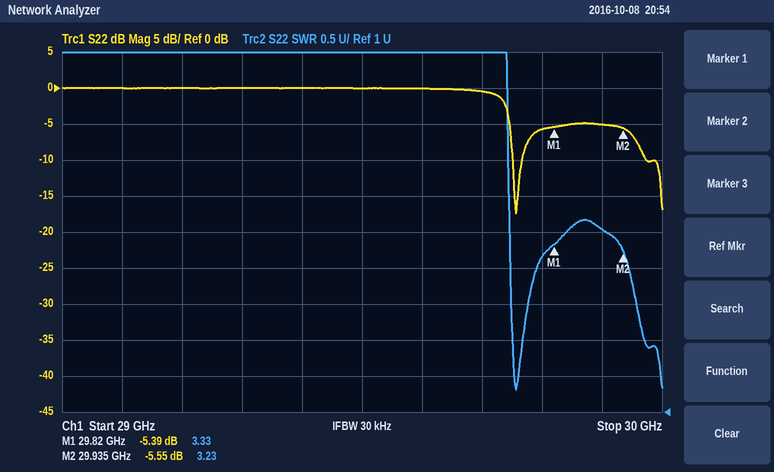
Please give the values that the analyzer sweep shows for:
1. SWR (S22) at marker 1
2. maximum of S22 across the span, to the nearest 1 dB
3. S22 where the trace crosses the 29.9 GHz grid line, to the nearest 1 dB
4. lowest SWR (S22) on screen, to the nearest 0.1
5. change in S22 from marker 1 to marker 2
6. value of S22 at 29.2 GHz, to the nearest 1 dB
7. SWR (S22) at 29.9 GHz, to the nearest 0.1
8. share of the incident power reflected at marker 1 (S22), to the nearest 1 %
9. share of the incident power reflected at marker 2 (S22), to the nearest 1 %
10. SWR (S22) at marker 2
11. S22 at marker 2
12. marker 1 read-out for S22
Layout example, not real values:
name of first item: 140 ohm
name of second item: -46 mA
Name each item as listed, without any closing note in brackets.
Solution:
SWR (S22) at marker 1: 3.33
maximum of S22 across the span, to the nearest 1 dB: 0 dB
S22 where the trace crosses the 29.9 GHz grid line, to the nearest 1 dB: -5 dB
lowest SWR (S22) on screen, to the nearest 0.1: 1.3
change in S22 from marker 1 to marker 2: -0.16 dB
value of S22 at 29.2 GHz, to the nearest 1 dB: 0 dB
SWR (S22) at 29.9 GHz, to the nearest 0.1: 3.5
share of the incident power reflected at marker 1 (S22), to the nearest 1 %: 29 %
share of the incident power reflected at marker 2 (S22), to the nearest 1 %: 28 %
SWR (S22) at marker 2: 3.23
S22 at marker 2: -5.55 dB
marker 1 read-out for S22: -5.39 dB
